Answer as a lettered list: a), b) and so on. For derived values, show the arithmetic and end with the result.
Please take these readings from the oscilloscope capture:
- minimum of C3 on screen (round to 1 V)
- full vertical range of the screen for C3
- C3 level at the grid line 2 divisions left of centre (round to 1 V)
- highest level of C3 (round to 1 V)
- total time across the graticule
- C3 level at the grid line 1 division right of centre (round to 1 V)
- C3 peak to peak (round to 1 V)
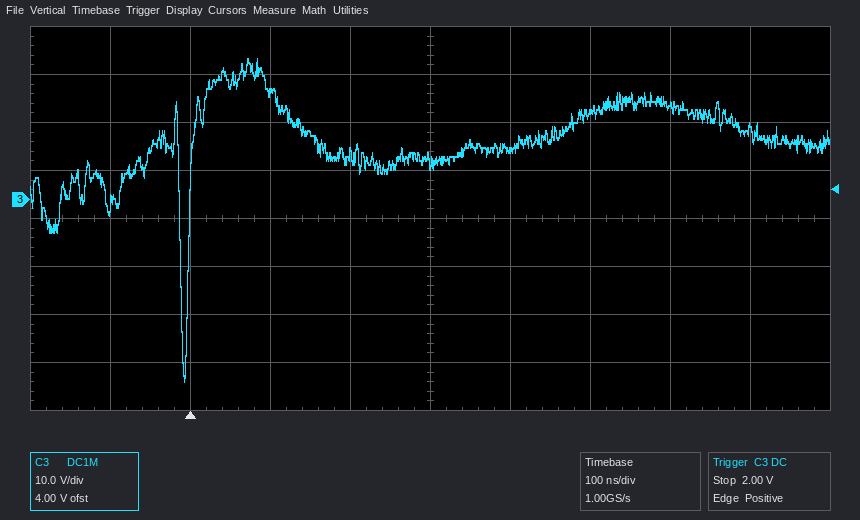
a) -38 V
b) 80 V
c) 22 V
d) 29 V
e) 1 µs
f) 10 V
g) 29 V − (-38 V) = 67 V
